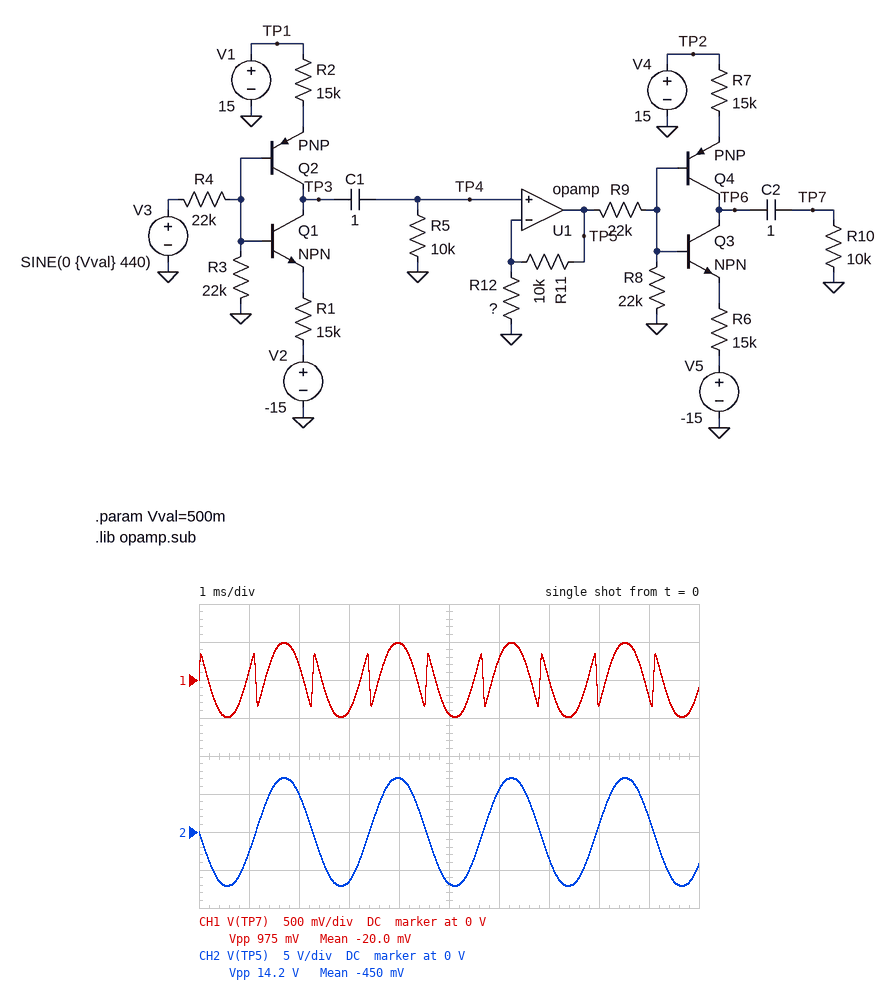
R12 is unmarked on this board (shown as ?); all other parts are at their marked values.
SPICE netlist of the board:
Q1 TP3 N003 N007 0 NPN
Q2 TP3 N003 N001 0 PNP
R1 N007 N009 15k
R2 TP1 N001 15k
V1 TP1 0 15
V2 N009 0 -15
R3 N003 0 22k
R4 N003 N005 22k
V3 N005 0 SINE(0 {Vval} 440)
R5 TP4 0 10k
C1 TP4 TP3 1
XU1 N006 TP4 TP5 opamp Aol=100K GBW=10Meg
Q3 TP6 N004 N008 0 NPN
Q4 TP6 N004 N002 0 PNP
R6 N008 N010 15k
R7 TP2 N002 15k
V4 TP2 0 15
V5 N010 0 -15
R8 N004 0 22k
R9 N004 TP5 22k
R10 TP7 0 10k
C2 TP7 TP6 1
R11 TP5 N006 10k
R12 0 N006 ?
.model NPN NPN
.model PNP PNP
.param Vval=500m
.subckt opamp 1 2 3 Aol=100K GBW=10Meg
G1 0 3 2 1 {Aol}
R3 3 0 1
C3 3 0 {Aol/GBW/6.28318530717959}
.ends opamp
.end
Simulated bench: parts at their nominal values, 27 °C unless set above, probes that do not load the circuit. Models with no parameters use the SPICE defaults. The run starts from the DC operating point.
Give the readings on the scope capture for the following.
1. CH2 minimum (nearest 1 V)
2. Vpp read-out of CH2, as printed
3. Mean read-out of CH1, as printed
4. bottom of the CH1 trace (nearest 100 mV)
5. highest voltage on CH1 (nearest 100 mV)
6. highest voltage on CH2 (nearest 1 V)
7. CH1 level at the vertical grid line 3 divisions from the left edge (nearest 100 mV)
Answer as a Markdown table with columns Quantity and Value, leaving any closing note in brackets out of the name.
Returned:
| Quantity | Value |
|---|---|
| CH2 minimum | -7 V |
| Vpp read-out of CH2, as printed | 14.2 V |
| Mean read-out of CH1, as printed | -20.0 mV |
| bottom of the CH1 trace | -500 mV |
| highest voltage on CH1 | 500 mV |
| highest voltage on CH2 | 7 V |
| CH1 level at the vertical grid line 3 divisions from the left edge | -400 mV |
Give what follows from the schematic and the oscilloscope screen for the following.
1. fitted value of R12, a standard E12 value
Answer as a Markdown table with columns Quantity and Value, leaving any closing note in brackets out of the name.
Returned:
| Quantity | Value |
|---|---|
| fitted value of R12, a standard E12 value | 470 Ω |
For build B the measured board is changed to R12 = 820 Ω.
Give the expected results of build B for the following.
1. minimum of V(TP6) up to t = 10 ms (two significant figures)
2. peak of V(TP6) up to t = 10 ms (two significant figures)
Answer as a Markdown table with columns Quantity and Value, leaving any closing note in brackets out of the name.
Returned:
| Quantity | Value |
|---|---|
| minimum of V(TP6) up to t = 10 ms | -340 mV |
| peak of V(TP6) up to t = 10 ms | 340 mV |
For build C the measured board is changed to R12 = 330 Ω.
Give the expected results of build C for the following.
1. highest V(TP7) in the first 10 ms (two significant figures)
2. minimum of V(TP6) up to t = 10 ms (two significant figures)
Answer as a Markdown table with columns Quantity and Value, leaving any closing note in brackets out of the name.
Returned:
| Quantity | Value |
|---|---|
| highest V(TP7) in the first 10 ms | 880 mV |
| minimum of V(TP6) up to t = 10 ms | -880 mV |
